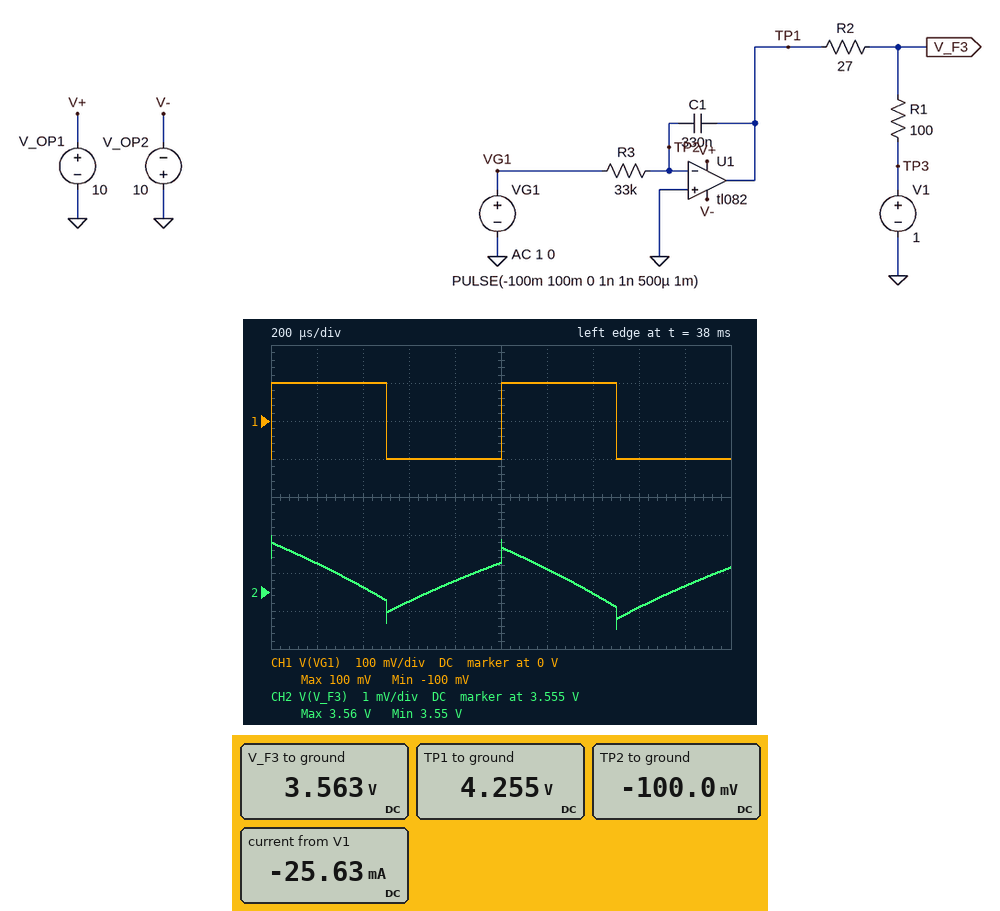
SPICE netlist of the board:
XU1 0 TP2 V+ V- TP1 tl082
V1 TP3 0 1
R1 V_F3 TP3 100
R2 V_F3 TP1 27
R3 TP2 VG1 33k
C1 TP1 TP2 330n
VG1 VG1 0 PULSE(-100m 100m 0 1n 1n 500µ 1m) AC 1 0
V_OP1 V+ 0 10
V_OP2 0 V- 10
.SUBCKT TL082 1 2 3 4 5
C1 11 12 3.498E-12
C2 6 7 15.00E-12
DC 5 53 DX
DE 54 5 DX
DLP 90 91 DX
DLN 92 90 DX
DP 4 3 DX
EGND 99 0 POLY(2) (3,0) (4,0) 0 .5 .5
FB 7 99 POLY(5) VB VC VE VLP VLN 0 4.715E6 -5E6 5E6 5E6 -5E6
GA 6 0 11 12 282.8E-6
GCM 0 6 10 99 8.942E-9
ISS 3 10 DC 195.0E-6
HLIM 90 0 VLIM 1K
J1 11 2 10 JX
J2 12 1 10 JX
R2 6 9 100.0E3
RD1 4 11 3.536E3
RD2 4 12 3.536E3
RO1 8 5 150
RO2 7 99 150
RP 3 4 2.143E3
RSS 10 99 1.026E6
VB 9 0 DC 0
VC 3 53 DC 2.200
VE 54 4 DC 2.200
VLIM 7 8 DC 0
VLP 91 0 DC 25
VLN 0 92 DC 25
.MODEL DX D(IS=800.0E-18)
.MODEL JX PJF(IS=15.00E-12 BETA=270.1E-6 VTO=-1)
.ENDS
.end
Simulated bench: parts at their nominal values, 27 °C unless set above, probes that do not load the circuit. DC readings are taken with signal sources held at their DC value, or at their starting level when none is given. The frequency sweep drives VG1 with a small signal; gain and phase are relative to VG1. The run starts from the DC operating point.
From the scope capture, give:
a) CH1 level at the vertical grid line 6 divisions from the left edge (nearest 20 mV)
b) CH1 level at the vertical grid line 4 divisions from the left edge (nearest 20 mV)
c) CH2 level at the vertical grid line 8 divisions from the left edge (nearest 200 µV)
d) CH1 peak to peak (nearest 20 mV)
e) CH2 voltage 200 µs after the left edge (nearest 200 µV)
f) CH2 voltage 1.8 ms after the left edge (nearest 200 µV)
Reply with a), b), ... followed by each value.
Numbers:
a) 100 mV
b) -100 mV
c) 3.5546 V
d) 200 mV
e) 3.5558 V
f) 3.5552 V
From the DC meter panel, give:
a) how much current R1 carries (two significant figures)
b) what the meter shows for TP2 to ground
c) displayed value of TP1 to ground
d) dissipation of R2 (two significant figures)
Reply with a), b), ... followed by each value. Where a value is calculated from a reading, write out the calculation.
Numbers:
a) (3.563 V - 1 V) / 100 Ω = 26 mA
b) -100.0 mV
c) 4.255 V
d) (4.255 V - 3.563 V)^2 / 27 Ω = 18 mW
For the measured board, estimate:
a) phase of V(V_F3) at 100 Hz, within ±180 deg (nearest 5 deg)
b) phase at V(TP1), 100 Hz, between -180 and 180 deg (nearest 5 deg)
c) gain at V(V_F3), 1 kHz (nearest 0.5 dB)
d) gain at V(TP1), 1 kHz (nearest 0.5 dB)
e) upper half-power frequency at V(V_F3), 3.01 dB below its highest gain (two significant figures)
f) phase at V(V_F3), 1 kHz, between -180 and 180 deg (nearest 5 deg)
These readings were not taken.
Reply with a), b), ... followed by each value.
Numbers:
a) 60 deg
b) 60 deg
c) -50.5 dB
d) -48.5 dB
e) 14 Hz
f) 10 deg
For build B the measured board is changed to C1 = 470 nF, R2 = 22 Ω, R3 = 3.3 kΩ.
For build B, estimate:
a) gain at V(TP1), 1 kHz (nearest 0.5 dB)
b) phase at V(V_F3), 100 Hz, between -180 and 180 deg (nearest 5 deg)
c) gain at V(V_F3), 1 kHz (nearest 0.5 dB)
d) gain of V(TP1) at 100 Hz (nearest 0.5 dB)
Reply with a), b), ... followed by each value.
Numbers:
a) -29.0 dB
b) 85 deg
c) -31.0 dB
d) -29.5 dB
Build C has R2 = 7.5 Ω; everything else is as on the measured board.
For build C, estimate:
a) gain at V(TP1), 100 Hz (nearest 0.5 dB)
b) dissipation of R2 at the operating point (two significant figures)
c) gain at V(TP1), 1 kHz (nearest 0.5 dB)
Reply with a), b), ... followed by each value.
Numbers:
a) -46.0 dB
b) 4.9 mW
c) -50.0 dB
